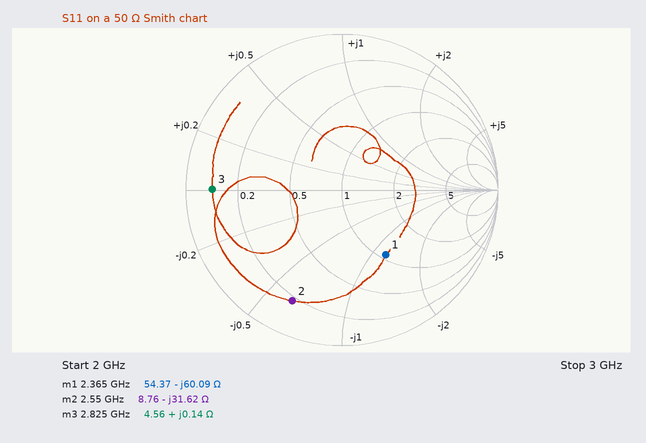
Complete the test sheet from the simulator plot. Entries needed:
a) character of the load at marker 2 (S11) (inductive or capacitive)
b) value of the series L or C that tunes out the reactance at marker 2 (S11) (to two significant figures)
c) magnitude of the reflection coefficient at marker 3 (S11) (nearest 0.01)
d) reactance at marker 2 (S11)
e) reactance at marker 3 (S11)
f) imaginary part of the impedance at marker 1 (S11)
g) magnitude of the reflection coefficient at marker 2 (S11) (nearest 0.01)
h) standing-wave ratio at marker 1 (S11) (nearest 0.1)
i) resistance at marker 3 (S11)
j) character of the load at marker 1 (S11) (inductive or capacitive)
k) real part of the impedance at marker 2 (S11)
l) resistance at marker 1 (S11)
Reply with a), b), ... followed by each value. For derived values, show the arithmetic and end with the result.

a) capacitive
b) L = 31.62 Ω/(2π × 2.55 GHz) ≈ 2.0 nH
c) 0.83
d) -31.62 Ω
e) +0.14 Ω
f) -60.09 Ω
g) 0.78
h) 3.0
i) 4.56 Ω
j) capacitive
k) 8.76 Ω
l) 54.37 Ω
